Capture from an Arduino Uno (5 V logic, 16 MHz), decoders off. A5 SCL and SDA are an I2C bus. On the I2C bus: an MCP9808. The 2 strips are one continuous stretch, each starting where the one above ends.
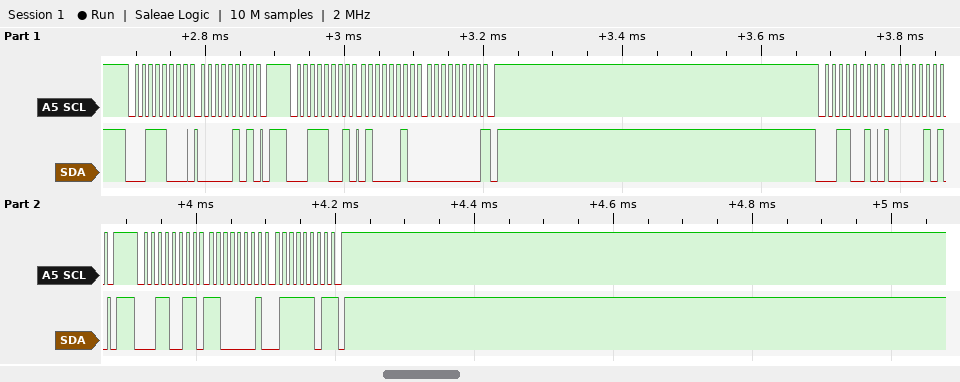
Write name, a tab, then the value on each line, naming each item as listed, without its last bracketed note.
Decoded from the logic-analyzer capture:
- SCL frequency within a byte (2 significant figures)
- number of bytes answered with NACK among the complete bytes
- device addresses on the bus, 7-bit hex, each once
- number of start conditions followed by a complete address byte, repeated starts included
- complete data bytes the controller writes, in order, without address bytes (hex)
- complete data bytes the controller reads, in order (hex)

SCL frequency within a byte	100 kHz
number of bytes answered with NACK among the complete bytes	2
device addresses on the bus, 7-bit hex, each once	0x1C 0x19
number of start conditions followed by a complete address byte, repeated starts included	4
complete data bytes the controller writes, in order, without address bytes	05 05
complete data bytes the controller reads, in order	42 00 C1 7D
